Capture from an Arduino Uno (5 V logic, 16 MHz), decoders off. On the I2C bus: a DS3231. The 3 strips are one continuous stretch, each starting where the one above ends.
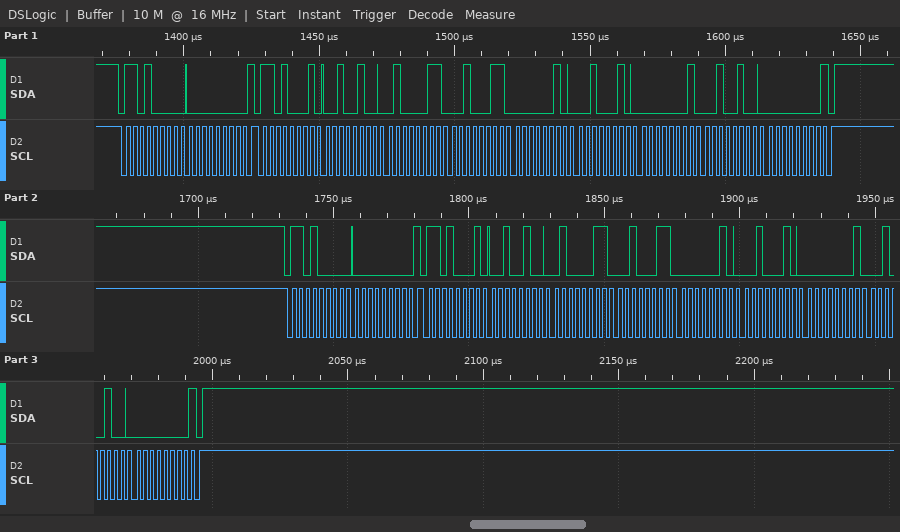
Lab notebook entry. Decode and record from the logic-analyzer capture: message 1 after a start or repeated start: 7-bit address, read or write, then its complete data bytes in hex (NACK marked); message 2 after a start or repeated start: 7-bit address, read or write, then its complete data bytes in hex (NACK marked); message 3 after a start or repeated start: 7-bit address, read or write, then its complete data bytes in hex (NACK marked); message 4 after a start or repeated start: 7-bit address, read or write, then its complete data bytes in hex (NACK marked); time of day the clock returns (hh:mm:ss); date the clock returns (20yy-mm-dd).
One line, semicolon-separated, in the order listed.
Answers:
0x68 write: 00; 0x68 read: 24 43 23 02 22 01 24 00 NACK; 0x68 write: 00; 0x68 read: 24 43 23 02 22 01 24 00 NACK; 23:43:24; 2024-01-22
